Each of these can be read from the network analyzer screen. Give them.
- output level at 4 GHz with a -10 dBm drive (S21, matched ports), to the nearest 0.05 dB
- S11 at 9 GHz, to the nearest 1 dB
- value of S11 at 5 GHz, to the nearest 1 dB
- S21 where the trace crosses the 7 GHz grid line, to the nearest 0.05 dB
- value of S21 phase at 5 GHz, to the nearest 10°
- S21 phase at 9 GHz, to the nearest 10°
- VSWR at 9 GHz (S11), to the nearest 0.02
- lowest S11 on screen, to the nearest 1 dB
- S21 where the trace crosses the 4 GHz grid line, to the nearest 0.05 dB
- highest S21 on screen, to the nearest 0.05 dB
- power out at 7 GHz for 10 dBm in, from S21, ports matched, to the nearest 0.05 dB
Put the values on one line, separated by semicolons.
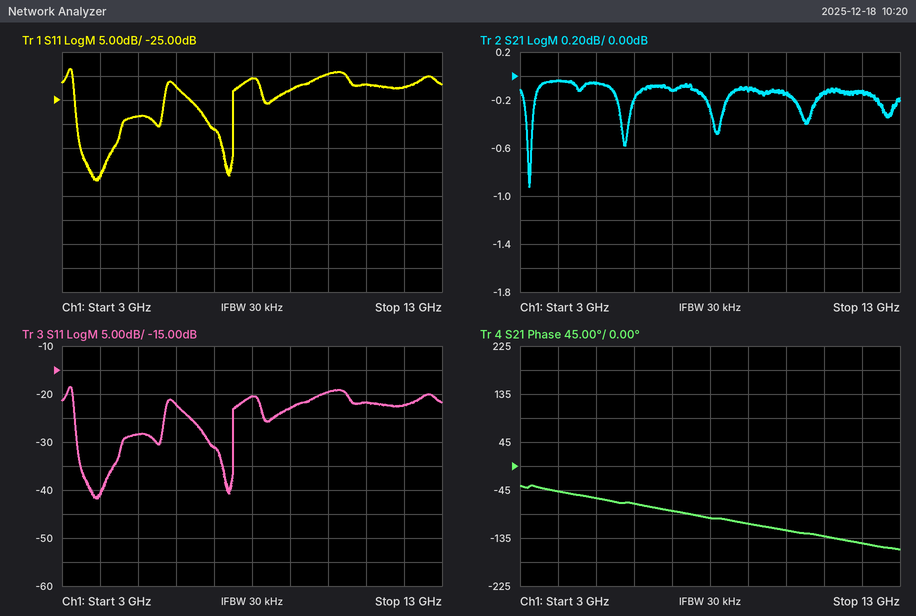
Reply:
-10.05 dBm; -23 dB; -28 dB; -0.10 dB; -60°; -110°; 1.16; -42 dB; -0.05 dB; -0.05 dB; 9.90 dBm
